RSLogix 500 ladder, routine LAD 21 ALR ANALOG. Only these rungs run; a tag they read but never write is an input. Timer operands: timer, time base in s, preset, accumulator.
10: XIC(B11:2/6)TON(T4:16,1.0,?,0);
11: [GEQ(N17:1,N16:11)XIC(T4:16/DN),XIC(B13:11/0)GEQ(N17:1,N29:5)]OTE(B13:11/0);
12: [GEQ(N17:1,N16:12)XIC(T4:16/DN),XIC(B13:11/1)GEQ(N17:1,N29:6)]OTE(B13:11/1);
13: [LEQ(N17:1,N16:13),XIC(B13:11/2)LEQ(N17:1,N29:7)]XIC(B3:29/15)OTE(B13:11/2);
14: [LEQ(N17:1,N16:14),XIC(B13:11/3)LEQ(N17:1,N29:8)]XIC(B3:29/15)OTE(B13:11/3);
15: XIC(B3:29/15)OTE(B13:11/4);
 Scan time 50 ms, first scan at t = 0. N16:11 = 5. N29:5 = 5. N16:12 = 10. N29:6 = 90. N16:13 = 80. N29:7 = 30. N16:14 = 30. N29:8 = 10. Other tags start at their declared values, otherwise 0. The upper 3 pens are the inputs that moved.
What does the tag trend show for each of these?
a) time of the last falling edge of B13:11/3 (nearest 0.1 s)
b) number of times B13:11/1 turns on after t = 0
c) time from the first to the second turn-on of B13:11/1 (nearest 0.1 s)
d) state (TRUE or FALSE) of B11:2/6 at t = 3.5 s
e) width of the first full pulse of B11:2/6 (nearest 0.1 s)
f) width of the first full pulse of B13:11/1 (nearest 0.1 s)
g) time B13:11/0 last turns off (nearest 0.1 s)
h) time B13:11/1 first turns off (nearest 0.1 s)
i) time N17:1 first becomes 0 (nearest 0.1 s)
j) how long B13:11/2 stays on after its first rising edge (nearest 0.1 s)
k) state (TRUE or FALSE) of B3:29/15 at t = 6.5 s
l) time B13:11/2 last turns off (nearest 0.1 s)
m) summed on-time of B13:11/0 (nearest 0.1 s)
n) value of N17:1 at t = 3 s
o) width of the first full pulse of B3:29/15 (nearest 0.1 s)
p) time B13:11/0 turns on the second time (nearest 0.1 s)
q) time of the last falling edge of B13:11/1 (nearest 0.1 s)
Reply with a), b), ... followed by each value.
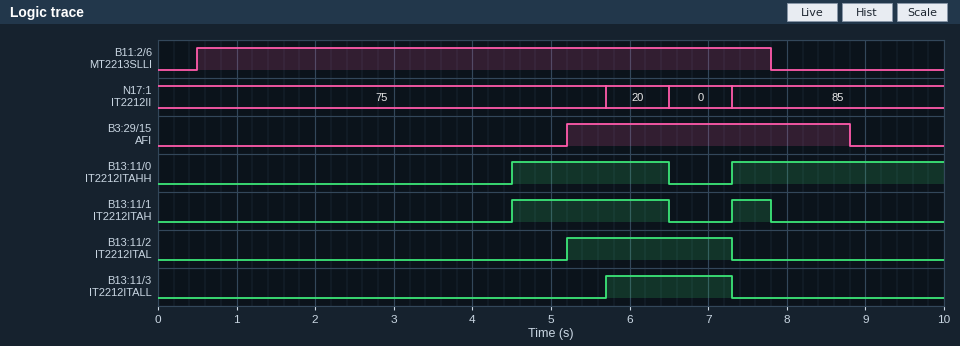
a) 7.3 s
b) 2
c) 2.8 s
d) TRUE
e) 7.3 s
f) 2.0 s
g) 6.5 s
h) 6.5 s
i) 6.5 s
j) 2.1 s
k) TRUE
l) 7.3 s
m) 4.7 s
n) 75
o) 3.6 s
p) 7.3 s
q) 7.8 s
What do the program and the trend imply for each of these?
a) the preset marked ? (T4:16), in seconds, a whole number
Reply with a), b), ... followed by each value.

a) 4 s
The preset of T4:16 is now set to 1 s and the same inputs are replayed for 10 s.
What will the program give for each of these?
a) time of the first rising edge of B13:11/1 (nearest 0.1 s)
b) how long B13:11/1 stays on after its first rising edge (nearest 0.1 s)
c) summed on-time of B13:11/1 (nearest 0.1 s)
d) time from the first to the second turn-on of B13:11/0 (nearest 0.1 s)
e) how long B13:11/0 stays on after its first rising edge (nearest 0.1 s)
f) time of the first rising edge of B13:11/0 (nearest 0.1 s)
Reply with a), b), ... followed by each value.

a) 1.5 s
b) 5.0 s
c) 5.5 s
d) 5.8 s
e) 5.0 s
f) 1.5 s
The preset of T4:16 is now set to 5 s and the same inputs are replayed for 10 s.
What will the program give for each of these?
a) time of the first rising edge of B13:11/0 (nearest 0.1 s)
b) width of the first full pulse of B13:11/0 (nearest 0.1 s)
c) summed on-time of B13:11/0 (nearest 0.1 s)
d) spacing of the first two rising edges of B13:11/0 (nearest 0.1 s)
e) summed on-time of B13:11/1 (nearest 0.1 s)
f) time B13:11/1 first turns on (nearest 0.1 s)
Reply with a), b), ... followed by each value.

a) 5.5 s
b) 1.0 s
c) 3.7 s
d) 1.8 s
e) 1.5 s
f) 5.5 s
